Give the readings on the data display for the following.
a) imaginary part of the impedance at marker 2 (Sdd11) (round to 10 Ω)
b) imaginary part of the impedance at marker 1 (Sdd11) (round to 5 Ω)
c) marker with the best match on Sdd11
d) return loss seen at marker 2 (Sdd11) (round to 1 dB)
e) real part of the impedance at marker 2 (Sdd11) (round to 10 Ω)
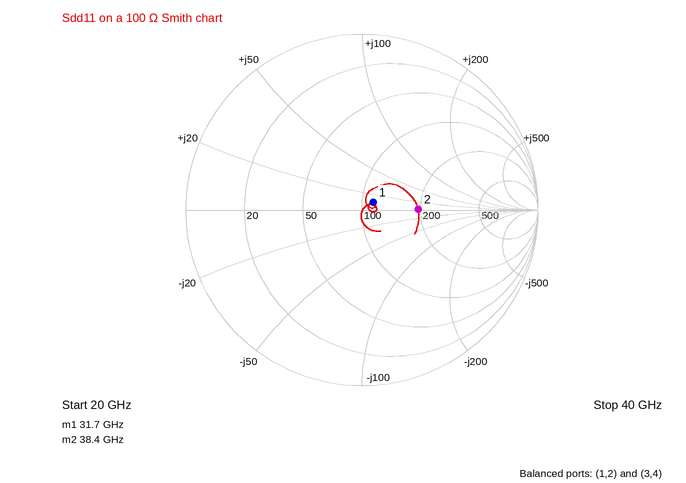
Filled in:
0 Ω
+10 Ω
marker 1
10 dB
190 Ω
